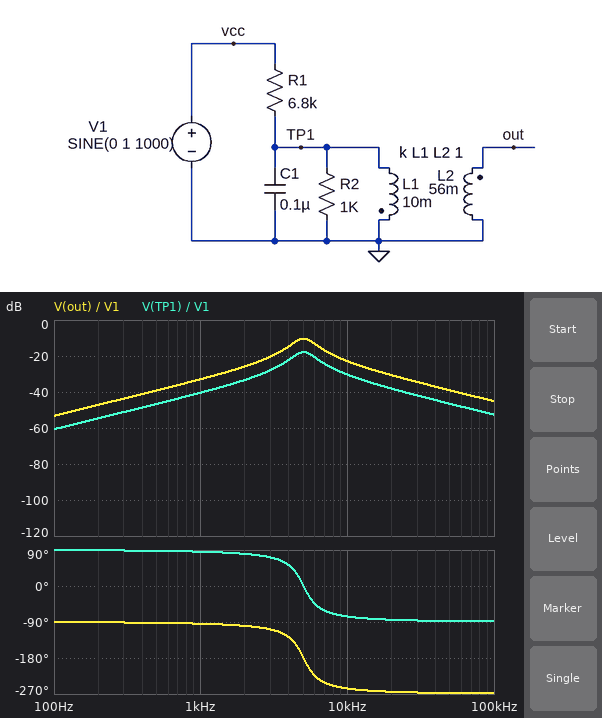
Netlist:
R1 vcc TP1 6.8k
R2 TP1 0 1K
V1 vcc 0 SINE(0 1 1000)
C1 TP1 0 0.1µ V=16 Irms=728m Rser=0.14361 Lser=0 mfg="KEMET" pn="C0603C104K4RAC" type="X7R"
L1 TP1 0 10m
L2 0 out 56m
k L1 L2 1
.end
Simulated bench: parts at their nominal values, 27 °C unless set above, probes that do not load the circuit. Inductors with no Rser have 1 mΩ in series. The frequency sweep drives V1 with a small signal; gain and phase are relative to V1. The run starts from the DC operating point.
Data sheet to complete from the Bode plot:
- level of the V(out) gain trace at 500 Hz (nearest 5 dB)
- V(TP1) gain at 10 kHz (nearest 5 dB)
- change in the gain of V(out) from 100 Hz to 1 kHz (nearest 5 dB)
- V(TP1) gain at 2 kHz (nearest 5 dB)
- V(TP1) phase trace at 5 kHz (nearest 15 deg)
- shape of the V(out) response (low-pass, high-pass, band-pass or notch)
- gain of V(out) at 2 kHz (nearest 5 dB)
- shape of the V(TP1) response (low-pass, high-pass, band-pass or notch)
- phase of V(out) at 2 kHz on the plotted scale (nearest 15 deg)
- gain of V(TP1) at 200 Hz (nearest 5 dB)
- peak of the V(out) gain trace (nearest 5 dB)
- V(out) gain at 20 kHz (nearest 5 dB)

-40 dB
-30 dB
20 dB
-35 dB
0 deg
band-pass
-25 dB
band-pass
-105 deg
-55 dB
-10 dB
-30 dB
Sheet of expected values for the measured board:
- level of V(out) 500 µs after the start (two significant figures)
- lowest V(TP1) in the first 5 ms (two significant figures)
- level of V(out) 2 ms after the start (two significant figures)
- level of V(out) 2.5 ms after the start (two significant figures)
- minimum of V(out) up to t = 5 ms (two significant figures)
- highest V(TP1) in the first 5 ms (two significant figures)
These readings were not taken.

21 mV
-9.6 mV
-23 mV
23 mV
-32 mV
14 mV
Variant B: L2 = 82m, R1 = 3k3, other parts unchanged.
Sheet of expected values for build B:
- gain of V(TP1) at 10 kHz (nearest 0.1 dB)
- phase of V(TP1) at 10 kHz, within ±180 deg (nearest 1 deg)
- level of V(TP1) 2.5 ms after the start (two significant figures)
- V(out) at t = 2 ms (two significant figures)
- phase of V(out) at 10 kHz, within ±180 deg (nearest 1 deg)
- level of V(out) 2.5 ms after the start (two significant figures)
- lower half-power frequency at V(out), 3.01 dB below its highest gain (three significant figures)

-24.1 dB
-74 deg
-20 mV
-56 mV
106 deg
56 mV
4.10 kHz
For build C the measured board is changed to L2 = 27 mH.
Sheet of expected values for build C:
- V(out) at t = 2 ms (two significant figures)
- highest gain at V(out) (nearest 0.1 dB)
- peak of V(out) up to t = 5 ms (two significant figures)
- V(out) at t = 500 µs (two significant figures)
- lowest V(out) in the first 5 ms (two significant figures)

-16 mV
-13.5 dB
16 mV
15 mV
-22 mV
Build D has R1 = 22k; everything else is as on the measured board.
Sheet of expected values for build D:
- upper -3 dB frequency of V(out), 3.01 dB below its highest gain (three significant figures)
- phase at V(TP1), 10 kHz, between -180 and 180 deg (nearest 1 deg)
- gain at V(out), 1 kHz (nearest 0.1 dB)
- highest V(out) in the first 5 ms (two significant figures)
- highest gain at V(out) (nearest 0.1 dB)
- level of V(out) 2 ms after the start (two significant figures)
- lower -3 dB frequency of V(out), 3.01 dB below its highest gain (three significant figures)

5.93 kHz
-77 deg
-43.1 dB
7.0 mV
-19.8 dB
-7.0 mV
4.27 kHz
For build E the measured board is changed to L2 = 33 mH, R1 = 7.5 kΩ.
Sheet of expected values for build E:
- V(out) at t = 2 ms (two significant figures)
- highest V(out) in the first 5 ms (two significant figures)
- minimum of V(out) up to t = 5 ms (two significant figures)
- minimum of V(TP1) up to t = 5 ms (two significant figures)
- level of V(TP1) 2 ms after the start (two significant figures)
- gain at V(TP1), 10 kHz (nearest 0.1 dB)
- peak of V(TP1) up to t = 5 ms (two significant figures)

-16 mV
16 mV
-22 mV
-8.7 mV
8.7 mV
-31.2 dB
12 mV
